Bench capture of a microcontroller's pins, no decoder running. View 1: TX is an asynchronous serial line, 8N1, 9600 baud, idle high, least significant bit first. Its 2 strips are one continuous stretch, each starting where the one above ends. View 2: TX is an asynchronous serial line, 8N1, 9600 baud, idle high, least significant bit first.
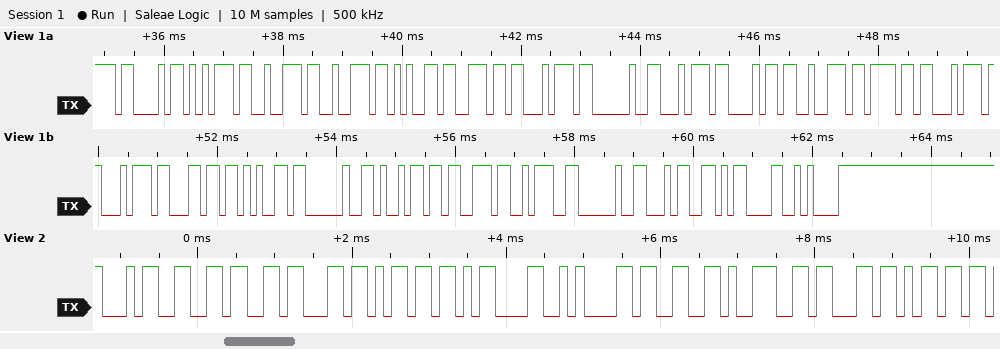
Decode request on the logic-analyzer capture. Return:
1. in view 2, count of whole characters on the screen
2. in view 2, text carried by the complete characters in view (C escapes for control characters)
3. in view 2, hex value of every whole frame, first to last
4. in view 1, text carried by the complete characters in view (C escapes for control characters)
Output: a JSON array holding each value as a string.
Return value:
["10", "\"46cm\\r\\n39cm\"", "34 36 63 6D 0D 0A 33 39 63 6D", "\"Current throttle is: 4\\r\\n\""]
